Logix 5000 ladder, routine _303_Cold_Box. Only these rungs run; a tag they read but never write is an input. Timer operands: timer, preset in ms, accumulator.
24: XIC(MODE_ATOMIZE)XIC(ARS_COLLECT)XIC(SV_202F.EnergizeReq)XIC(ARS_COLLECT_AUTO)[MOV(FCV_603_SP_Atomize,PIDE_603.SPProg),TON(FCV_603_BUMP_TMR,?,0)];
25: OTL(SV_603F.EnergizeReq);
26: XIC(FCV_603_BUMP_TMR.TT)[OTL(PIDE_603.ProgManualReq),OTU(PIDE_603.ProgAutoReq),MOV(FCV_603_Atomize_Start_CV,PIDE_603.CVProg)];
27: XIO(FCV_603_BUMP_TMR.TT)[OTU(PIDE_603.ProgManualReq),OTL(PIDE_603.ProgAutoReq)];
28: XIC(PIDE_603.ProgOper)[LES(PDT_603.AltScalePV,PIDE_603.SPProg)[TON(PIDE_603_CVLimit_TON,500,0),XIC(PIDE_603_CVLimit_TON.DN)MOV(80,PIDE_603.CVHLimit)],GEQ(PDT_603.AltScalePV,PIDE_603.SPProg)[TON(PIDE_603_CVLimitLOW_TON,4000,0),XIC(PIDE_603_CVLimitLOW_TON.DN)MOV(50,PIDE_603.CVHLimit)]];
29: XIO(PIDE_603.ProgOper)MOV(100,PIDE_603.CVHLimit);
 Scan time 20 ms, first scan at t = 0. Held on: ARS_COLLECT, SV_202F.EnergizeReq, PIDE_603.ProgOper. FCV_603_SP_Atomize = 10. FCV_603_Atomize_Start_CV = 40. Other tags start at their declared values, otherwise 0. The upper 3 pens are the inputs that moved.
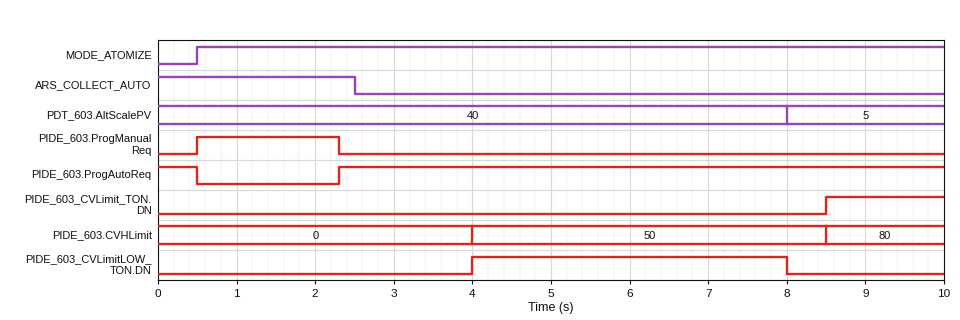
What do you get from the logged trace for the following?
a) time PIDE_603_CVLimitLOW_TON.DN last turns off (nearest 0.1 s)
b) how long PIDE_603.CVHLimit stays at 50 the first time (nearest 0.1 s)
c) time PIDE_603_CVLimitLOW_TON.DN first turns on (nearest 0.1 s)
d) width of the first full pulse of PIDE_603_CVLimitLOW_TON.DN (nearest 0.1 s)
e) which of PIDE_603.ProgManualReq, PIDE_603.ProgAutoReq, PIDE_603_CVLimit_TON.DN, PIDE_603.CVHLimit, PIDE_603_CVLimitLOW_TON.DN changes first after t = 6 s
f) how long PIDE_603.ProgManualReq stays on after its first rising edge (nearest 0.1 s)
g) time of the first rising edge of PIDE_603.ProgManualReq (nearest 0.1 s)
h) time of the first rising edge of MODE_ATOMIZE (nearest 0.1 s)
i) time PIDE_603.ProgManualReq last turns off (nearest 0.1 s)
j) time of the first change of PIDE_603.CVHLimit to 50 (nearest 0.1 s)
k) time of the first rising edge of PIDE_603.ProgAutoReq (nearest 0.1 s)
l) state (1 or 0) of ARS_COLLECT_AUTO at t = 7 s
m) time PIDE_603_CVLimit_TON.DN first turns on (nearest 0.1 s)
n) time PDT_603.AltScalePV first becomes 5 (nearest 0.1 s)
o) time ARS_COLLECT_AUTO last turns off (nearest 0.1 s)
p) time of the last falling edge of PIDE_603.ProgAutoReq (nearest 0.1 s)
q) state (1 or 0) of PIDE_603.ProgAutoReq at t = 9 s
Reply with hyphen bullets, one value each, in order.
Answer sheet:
- 8.0 s
- 4.5 s
- 4.0 s
- 4.0 s
- PIDE_603_CVLimitLOW_TON.DN
- 1.8 s
- 0.5 s
- 0.5 s
- 2.3 s
- 4.0 s
- 2.3 s
- 0
- 8.5 s
- 8.0 s
- 2.5 s
- 0.5 s
- 1
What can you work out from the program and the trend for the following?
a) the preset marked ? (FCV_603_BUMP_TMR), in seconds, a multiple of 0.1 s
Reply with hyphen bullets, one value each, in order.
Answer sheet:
- 1.8 s
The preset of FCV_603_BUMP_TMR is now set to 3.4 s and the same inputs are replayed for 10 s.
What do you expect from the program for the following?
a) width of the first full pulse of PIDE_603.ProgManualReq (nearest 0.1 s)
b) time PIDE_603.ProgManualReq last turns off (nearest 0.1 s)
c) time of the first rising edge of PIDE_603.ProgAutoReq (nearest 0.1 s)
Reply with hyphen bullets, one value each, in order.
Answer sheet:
- 2.0 s
- 2.5 s
- 2.5 s
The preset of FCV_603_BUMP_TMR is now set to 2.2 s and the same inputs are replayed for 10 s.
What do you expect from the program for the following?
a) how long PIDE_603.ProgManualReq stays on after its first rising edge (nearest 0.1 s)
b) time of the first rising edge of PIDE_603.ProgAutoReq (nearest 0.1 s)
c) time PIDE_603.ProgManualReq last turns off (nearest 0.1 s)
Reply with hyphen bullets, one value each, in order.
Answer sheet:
- 2.0 s
- 2.5 s
- 2.5 s
